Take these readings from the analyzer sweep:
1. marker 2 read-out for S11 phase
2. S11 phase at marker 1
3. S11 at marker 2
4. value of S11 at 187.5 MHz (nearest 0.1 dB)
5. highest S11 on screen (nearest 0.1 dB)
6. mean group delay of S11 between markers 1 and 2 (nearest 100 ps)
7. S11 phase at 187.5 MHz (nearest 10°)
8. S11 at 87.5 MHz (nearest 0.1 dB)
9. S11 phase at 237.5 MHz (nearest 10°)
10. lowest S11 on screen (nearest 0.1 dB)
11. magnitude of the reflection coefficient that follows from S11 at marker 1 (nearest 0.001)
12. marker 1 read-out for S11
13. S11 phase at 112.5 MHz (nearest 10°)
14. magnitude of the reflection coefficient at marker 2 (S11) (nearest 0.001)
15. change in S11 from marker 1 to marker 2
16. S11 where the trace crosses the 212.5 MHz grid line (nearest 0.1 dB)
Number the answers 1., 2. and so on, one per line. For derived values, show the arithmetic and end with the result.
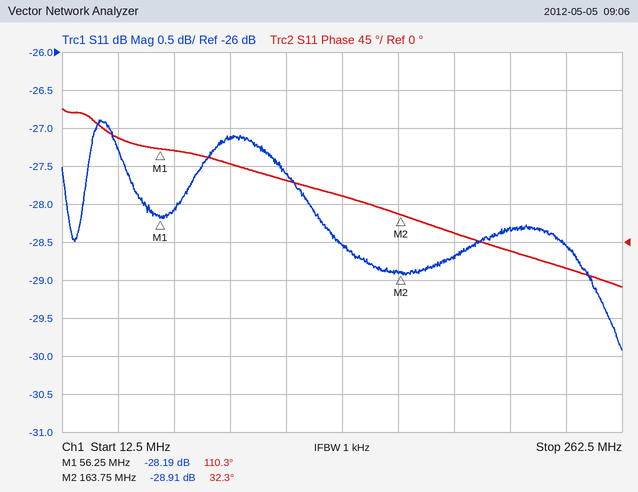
1. 32.3°
2. 110.3°
3. -28.91 dB
4. -28.7 dB
5. -26.9 dB
6. −(32.3° − (110.3°))/(360° × 107.5 MHz) ≈ 2.0 ns
7. 10°
8. -27.1 dB
9. -30°
10. -29.9 dB
11. 10^(-28.19/20) ≈ 0.039
12. -28.19 dB
13. 70°
14. 10^(-28.91/20) ≈ 0.036
15. -28.91 − (-28.19) = -0.72 dB
16. -28.3 dB
